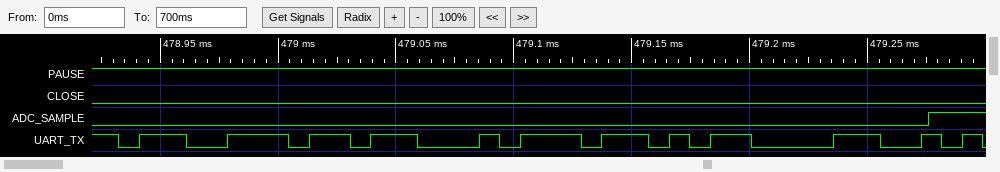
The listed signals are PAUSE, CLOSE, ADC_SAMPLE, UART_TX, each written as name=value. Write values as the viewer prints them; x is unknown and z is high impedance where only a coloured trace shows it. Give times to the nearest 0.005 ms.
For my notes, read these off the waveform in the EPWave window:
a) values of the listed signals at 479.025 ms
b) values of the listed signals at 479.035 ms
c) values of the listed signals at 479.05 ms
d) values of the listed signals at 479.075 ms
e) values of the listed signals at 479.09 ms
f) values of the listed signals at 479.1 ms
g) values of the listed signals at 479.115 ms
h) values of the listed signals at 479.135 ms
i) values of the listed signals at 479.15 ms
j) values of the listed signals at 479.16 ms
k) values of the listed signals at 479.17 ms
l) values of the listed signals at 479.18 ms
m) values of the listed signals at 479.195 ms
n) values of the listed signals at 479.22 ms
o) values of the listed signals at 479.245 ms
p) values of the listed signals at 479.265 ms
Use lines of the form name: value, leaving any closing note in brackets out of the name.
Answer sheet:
values of the listed signals at 479.025 ms: PAUSE=1, CLOSE=0, ADC_SAMPLE=0, UART_TX=1
values of the listed signals at 479.035 ms: PAUSE=1, CLOSE=0, ADC_SAMPLE=0, UART_TX=0
values of the listed signals at 479.05 ms: PAUSE=1, CLOSE=0, ADC_SAMPLE=0, UART_TX=1
values of the listed signals at 479.075 ms: PAUSE=1, CLOSE=0, ADC_SAMPLE=0, UART_TX=0
values of the listed signals at 479.09 ms: PAUSE=1, CLOSE=0, ADC_SAMPLE=0, UART_TX=1
values of the listed signals at 479.1 ms: PAUSE=1, CLOSE=0, ADC_SAMPLE=0, UART_TX=0
values of the listed signals at 479.115 ms: PAUSE=1, CLOSE=0, ADC_SAMPLE=0, UART_TX=1
values of the listed signals at 479.135 ms: PAUSE=1, CLOSE=0, ADC_SAMPLE=0, UART_TX=0
values of the listed signals at 479.15 ms: PAUSE=1, CLOSE=0, ADC_SAMPLE=0, UART_TX=1
values of the listed signals at 479.16 ms: PAUSE=1, CLOSE=0, ADC_SAMPLE=0, UART_TX=0
values of the listed signals at 479.17 ms: PAUSE=1, CLOSE=0, ADC_SAMPLE=0, UART_TX=1
values of the listed signals at 479.18 ms: PAUSE=1, CLOSE=0, ADC_SAMPLE=0, UART_TX=0
values of the listed signals at 479.195 ms: PAUSE=1, CLOSE=0, ADC_SAMPLE=0, UART_TX=1
values of the listed signals at 479.22 ms: PAUSE=1, CLOSE=0, ADC_SAMPLE=0, UART_TX=0
values of the listed signals at 479.245 ms: PAUSE=1, CLOSE=0, ADC_SAMPLE=0, UART_TX=1
values of the listed signals at 479.265 ms: PAUSE=1, CLOSE=0, ADC_SAMPLE=0, UART_TX=0
